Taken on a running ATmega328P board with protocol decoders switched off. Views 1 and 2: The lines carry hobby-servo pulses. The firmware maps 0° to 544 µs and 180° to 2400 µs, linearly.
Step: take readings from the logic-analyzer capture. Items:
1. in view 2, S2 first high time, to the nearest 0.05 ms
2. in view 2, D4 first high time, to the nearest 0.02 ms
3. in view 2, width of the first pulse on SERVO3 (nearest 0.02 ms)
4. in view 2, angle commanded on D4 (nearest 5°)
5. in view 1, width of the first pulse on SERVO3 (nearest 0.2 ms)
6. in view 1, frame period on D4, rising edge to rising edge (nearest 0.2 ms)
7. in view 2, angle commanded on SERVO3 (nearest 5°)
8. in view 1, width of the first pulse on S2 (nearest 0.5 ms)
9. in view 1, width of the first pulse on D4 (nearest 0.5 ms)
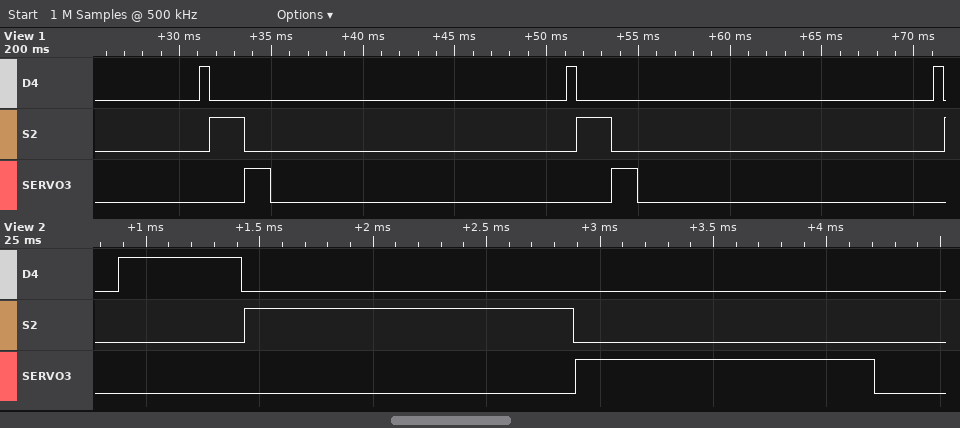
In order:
1.45 ms
0.54 ms
1.32 ms
0°
1.4 ms
20.0 ms
75°
2.0 ms
0.5 ms
